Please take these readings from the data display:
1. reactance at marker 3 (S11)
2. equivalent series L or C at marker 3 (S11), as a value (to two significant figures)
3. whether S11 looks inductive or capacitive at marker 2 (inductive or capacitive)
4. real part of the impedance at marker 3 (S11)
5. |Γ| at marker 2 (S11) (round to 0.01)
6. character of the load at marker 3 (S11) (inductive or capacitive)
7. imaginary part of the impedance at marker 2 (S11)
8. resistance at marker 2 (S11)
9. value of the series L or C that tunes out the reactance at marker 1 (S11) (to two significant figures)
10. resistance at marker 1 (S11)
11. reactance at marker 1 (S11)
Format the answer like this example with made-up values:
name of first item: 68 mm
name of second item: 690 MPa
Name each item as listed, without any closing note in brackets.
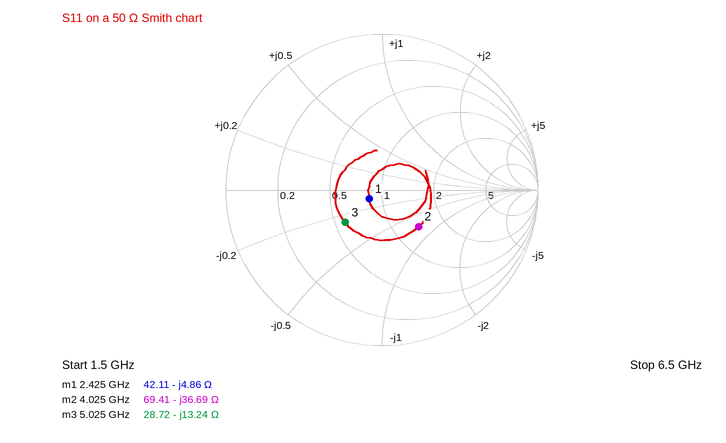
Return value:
reactance at marker 3: -13.24 Ω
equivalent series L or C at marker 3 (S11), as a value: 2.4 pF
whether S11 looks inductive or capacitive at marker 2: capacitive
real part of the impedance at marker 3: 28.72 Ω
|Γ| at marker 2 (S11): 0.33
character of the load at marker 3 (S11): capacitive
imaginary part of the impedance at marker 2: -36.69 Ω
resistance at marker 2: 69.41 Ω
value of the series L or C that tunes out the reactance at marker 1 (S11): 320 pH
resistance at marker 1: 42.11 Ω
reactance at marker 1: -4.86 Ω
